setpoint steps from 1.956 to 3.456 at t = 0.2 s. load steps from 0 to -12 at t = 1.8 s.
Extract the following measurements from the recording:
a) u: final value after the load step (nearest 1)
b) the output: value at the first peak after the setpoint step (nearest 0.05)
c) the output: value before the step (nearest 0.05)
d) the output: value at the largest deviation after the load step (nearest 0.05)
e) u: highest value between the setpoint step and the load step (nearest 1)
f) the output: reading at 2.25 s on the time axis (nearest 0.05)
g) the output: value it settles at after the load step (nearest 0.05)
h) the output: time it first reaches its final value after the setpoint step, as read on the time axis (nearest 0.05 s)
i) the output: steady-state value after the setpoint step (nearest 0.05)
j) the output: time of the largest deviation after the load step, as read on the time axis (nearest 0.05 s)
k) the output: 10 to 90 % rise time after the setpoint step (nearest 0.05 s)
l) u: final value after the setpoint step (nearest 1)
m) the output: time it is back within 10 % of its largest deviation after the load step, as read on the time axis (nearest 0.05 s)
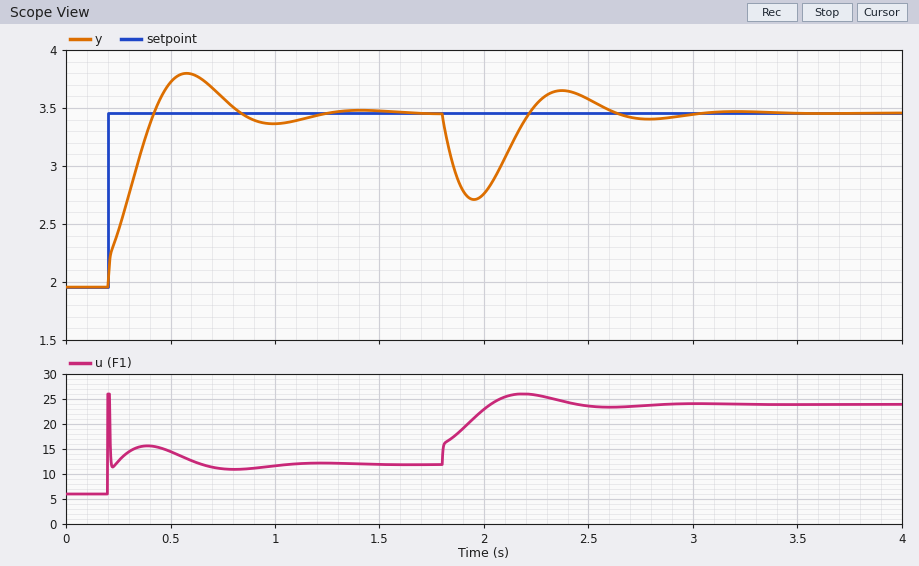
24
3.80
1.95
2.70
26
3.55
3.45
0.40 s
3.45
1.95 s
0.20 s
12
2.55 s
